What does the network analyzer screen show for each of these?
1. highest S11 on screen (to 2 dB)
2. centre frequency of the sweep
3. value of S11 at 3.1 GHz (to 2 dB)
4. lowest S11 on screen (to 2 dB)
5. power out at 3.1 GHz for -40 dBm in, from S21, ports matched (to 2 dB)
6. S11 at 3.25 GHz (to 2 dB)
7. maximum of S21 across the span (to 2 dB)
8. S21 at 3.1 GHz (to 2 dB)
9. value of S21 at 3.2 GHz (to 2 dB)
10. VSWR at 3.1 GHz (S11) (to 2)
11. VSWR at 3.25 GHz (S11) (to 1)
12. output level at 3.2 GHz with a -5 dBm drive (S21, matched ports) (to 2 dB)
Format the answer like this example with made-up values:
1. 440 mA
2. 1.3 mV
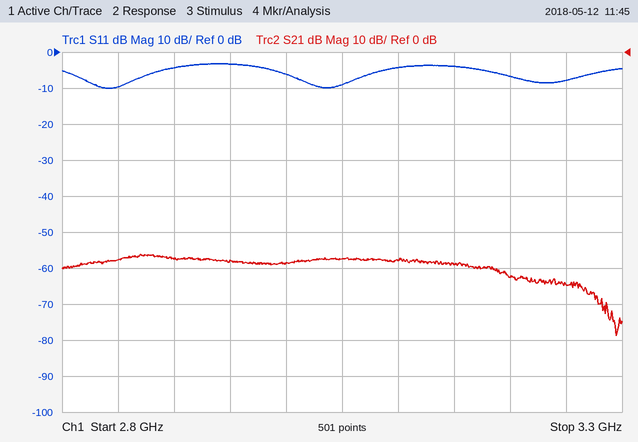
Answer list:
1. -4 dB
2. 3.05 GHz
3. -4 dB
4. -10 dB
5. -98 dBm
6. -8 dB
7. -56 dB
8. -58 dB
9. -62 dB
10. 4
11. 2
12. -68 dBm
